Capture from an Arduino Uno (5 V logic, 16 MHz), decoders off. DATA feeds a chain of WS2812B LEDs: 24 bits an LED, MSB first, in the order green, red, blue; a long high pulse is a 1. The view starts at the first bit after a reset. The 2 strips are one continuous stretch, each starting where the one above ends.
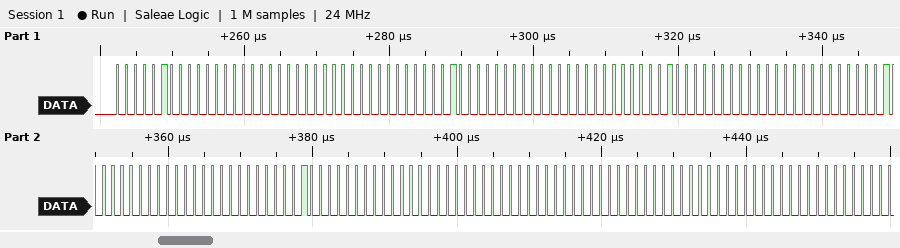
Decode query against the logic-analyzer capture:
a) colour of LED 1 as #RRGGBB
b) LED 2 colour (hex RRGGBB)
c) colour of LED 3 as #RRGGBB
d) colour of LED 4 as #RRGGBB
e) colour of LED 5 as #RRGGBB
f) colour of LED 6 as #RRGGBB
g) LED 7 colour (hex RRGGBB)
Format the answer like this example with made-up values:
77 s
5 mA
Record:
#000400
#040000
#040000
#040000
#040000
#000000
#000000
